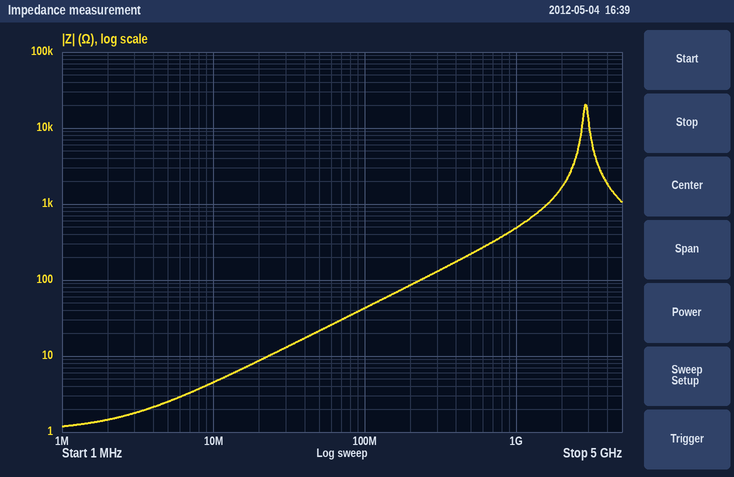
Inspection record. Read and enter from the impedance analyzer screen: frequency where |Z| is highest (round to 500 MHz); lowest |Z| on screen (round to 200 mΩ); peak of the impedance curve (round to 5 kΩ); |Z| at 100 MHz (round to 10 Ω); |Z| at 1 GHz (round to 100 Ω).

3.0 GHz
1.2 Ω
20 kΩ
40 Ω
500 Ω
